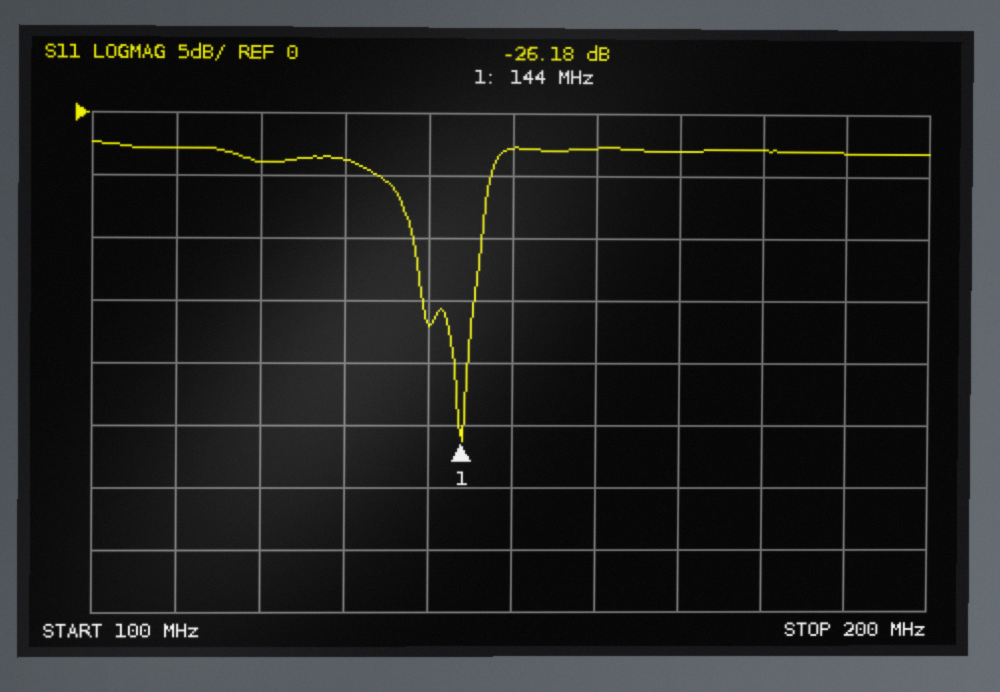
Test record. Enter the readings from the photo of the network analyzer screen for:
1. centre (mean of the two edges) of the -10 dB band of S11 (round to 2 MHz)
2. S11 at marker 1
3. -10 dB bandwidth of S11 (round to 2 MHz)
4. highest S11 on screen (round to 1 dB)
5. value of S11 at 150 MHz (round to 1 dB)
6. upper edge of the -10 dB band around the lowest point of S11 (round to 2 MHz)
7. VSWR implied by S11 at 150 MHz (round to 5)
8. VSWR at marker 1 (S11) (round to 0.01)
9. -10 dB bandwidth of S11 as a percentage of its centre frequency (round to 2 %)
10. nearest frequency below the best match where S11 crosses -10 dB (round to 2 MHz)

142 MHz
-26.18 dB
8 MHz
-2 dB
-3 dB
146 MHz
5
1.10
6 %
138 MHz
